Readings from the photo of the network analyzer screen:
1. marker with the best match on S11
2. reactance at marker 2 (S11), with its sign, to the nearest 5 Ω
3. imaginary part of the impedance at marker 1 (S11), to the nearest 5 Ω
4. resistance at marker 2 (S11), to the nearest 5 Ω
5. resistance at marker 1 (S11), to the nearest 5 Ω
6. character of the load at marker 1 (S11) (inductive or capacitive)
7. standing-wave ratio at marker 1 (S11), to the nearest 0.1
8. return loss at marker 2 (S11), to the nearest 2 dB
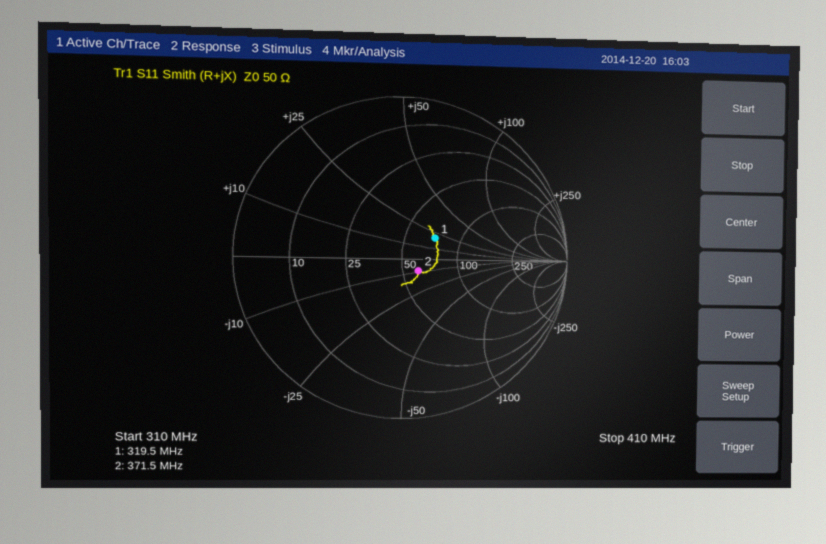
marker 2
-10 Ω
+20 Ω
60 Ω
70 Ω
inductive
1.6
18 dB
